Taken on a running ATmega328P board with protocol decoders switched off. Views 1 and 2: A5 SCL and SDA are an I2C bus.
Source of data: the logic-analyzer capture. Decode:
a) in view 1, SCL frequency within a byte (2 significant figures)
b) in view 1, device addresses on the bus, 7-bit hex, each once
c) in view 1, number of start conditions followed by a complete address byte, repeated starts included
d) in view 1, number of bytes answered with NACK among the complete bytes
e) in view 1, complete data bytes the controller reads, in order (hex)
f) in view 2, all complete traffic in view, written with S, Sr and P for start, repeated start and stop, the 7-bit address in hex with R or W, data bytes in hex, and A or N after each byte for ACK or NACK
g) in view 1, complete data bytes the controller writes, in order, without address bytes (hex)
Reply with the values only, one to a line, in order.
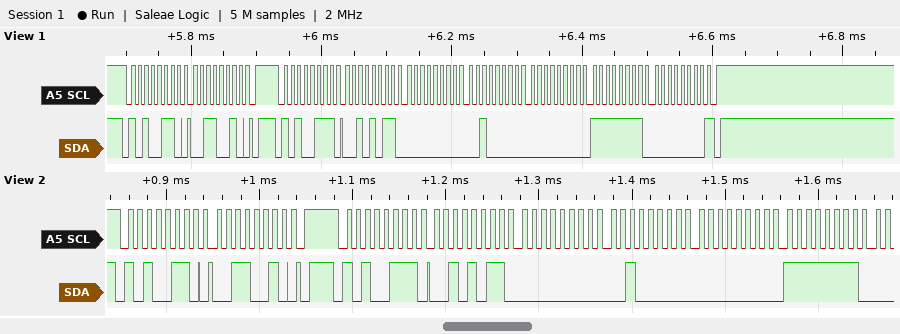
100 kHz
0x53
2
1
2B 00 20 00 FF 00
S 53W A 32 A P S 53R A 2B A 00 A 20 A 00 A FF A
32
